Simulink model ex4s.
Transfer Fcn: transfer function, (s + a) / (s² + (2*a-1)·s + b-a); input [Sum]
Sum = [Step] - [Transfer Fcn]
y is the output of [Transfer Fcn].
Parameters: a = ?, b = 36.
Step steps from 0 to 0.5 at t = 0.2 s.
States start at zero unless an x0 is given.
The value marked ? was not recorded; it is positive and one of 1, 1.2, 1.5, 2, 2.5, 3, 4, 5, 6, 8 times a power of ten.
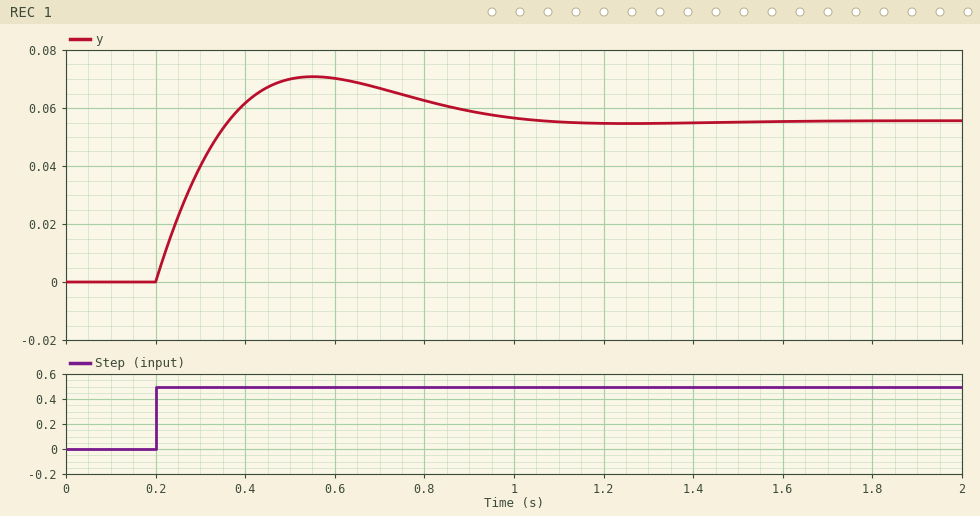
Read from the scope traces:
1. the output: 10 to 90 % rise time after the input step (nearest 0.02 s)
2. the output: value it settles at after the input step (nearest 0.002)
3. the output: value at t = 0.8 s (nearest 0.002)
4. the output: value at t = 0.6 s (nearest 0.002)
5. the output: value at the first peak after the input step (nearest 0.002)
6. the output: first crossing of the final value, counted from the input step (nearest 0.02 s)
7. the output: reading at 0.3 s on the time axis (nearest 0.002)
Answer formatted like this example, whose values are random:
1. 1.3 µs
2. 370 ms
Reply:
1. 0.12 s
2. 0.056
3. 0.062
4. 0.070
5. 0.070
6. 0.16 s
7. 0.040
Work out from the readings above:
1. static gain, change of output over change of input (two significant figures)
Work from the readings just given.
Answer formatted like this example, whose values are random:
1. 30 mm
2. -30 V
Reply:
1. 0.11
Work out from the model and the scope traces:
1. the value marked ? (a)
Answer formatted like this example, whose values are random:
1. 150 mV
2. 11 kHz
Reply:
1. 4
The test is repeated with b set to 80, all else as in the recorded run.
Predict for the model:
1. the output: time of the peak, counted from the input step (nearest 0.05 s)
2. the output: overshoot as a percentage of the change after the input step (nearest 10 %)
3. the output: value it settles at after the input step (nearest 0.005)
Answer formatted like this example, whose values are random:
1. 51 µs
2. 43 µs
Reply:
1. 0.20 s
2. 90 %
3. 0.025
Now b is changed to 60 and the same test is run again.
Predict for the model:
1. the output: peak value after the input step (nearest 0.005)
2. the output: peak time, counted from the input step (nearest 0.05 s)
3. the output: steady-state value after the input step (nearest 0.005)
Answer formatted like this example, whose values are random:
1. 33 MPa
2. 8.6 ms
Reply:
1. 0.055
2. 0.25 s
3. 0.035
